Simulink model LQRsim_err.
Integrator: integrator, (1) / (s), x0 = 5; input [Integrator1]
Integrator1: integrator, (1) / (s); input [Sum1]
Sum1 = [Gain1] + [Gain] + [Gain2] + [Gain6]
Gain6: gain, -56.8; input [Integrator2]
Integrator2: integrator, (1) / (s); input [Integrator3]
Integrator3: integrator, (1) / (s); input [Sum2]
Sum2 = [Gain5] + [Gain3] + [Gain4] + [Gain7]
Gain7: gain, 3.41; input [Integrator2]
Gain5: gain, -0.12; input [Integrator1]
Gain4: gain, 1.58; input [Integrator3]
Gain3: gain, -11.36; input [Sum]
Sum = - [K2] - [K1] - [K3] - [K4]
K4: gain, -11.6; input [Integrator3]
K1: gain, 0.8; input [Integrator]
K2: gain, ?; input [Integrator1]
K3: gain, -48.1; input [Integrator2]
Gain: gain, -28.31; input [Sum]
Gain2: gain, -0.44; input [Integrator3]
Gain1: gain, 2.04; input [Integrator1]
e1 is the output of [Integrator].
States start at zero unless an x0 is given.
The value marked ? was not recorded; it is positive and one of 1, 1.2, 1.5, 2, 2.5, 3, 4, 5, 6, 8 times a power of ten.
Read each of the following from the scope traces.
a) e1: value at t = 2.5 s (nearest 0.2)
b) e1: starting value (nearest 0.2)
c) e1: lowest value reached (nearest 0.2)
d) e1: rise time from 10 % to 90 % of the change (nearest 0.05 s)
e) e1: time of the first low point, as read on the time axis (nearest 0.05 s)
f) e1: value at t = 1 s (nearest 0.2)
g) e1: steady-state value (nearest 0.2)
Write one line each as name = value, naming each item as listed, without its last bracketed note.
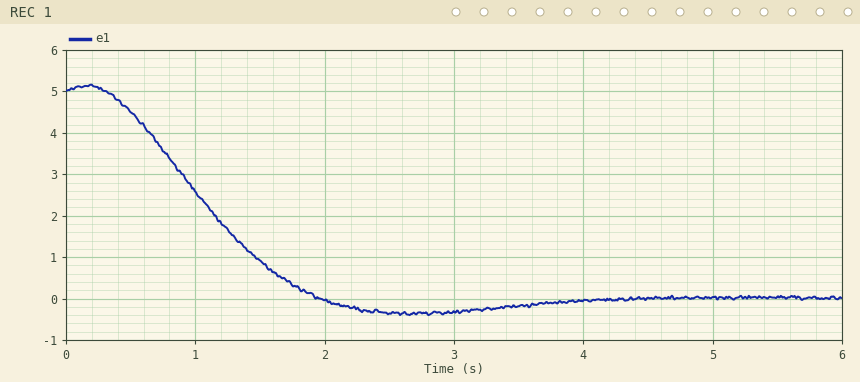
e1: value at t = 2.5 s = -0.4
e1: starting value = 5.0
e1: lowest value reached = -0.4
e1: rise time from 10 % to 90 % of the change = 1.15 s
e1: time of the first low point, as read on the time axis = 2.65 s
e1: value at t = 1 s = 2.6
e1: steady-state value = 0.0
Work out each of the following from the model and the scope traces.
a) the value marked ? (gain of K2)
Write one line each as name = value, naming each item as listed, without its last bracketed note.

the value marked ? = 2.5
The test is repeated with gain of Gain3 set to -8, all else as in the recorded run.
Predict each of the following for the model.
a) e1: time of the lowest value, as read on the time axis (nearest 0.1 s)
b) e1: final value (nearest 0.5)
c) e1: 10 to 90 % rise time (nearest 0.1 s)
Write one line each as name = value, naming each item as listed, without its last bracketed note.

e1: time of the lowest value, as read on the time axis = 3.0 s
e1: final value = 0.0
e1: 10 to 90 % rise time = 1.3 s
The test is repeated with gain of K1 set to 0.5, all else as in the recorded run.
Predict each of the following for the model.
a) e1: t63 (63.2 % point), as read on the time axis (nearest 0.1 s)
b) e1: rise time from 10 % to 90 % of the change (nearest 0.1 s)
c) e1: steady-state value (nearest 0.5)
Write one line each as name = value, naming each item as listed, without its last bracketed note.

e1: t63 (63.2 % point), as read on the time axis = 1.7 s
e1: rise time from 10 % to 90 % of the change = 2.2 s
e1: steady-state value = 0.0
